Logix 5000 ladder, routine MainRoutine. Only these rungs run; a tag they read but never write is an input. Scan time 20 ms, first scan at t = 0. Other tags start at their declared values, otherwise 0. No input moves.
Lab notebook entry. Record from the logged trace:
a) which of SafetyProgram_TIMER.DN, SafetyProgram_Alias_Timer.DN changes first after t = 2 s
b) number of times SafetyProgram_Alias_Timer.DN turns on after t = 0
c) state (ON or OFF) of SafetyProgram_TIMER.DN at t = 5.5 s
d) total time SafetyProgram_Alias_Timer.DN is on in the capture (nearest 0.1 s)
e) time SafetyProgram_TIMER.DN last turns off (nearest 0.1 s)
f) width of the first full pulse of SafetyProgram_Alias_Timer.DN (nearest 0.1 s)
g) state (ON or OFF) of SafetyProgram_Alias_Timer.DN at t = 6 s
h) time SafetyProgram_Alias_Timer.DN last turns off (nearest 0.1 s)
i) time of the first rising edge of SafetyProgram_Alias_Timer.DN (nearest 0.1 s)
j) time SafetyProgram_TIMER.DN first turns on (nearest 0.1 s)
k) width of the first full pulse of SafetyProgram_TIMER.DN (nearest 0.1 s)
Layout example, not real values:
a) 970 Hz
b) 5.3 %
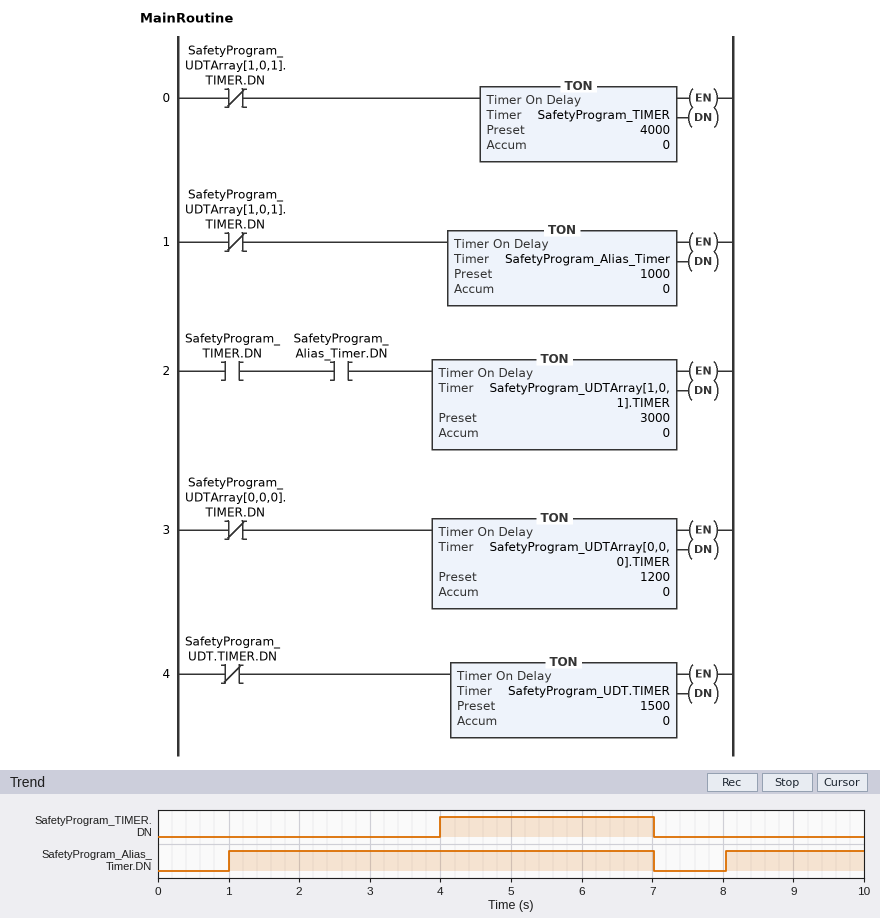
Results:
a) SafetyProgram_TIMER.DN
b) 2
c) ON
d) 8.0 s
e) 7.0 s
f) 6.0 s
g) ON
h) 7.0 s
i) 1.0 s
j) 4.0 s
k) 3.0 s
